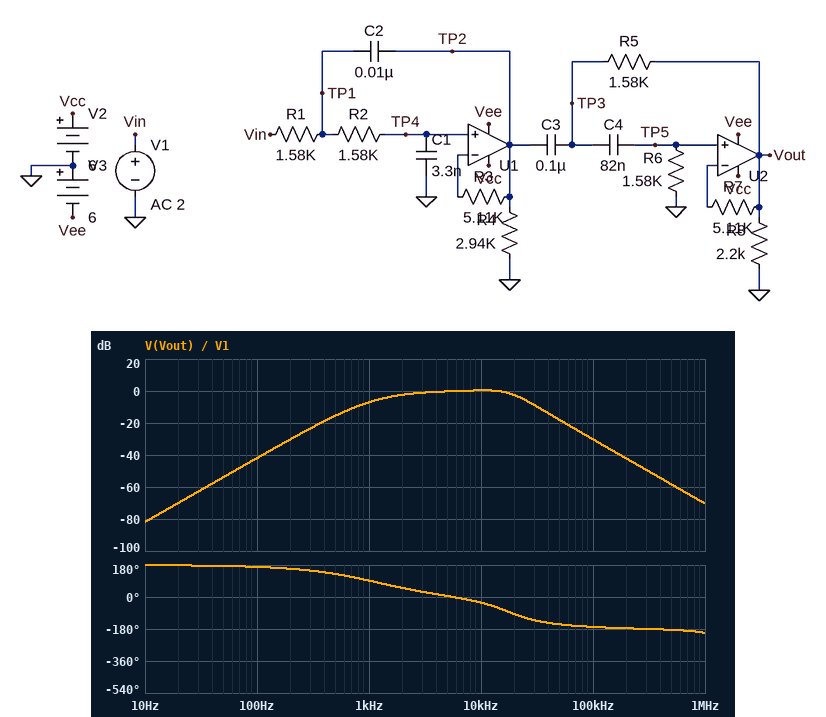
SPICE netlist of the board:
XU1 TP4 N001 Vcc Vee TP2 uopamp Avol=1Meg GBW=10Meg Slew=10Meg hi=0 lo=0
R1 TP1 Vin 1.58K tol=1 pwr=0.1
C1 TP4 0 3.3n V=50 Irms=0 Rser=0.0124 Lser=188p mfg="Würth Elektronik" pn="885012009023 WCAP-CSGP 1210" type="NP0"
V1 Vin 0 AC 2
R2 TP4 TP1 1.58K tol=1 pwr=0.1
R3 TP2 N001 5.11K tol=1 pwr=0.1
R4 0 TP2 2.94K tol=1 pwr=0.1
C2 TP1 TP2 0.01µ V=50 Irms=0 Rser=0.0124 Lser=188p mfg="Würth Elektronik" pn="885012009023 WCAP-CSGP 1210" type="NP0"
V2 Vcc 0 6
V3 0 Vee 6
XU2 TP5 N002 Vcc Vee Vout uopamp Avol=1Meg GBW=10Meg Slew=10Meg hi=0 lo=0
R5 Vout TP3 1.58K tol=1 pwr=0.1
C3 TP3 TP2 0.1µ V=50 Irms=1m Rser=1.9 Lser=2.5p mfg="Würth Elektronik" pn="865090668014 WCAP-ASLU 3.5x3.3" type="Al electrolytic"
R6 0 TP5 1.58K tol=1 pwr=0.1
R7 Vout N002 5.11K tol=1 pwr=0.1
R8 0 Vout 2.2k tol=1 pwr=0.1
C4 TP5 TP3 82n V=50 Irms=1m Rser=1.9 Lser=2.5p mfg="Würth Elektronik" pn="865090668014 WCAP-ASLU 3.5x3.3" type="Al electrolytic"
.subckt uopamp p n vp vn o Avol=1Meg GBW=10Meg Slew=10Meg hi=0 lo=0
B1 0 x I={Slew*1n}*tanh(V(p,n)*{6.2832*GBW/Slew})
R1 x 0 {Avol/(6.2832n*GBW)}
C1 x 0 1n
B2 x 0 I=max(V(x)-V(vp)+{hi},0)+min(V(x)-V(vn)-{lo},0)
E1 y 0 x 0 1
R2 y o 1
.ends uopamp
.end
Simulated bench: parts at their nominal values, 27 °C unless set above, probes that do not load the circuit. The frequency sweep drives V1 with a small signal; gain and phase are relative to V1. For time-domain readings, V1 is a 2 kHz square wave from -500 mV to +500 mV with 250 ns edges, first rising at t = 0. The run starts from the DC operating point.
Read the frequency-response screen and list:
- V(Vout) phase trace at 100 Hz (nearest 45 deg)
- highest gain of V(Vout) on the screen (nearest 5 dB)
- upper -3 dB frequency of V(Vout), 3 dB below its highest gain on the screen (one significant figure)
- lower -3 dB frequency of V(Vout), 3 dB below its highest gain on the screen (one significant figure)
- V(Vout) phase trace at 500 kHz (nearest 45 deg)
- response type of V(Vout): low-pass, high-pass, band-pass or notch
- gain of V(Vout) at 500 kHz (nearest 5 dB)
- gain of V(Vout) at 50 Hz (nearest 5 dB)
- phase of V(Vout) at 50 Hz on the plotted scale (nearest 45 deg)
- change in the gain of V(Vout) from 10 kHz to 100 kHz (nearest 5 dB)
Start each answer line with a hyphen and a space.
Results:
- 180 deg
- 0 dB
- 20 kHz
- 2 kHz
- -180 deg
- band-pass
- -60 dB
- -55 dB
- 180 deg
- -30 dB
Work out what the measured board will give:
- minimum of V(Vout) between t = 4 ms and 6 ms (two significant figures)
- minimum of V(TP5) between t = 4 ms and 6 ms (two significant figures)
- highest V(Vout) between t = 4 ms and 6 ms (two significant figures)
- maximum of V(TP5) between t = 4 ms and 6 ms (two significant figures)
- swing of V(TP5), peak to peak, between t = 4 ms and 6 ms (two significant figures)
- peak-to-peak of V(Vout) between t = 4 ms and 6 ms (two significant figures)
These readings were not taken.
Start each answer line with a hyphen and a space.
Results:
- -950 mV
- -950 mV
- 950 mV
- 950 mV
- 1.9 V
- 1.9 V
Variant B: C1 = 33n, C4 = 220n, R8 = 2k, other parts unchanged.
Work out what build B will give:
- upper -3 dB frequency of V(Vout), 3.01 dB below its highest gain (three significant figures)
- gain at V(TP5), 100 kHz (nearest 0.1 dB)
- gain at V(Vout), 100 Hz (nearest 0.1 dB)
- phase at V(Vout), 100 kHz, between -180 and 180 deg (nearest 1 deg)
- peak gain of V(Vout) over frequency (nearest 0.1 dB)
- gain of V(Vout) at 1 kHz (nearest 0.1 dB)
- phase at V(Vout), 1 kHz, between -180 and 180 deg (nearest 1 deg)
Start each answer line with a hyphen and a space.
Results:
- 3.34 kHz
- -50.4 dB
- -33.5 dB
- -169 deg
- -4.6 dB
- -5.2 dB
- 36 deg
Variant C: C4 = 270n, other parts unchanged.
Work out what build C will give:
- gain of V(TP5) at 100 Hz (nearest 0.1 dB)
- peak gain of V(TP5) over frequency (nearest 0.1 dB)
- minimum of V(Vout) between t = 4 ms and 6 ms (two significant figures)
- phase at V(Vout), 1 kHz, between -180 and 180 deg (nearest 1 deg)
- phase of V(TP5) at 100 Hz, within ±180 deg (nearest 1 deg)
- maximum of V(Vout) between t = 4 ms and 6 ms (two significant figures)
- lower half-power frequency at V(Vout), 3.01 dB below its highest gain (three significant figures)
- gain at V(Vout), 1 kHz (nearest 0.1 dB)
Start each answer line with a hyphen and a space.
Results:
- -31.8 dB
- 0.5 dB
- -910 mV
- 62 deg
- 159 deg
- 910 mV
- 1.25 kHz
- -3.6 dB
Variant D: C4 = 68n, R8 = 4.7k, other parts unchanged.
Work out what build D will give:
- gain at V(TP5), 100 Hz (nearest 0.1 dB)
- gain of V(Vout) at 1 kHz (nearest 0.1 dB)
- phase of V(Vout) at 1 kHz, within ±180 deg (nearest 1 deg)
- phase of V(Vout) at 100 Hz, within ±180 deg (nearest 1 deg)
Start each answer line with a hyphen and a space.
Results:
- -43.5 dB
- -8.1 dB
- 97 deg
- 170 deg
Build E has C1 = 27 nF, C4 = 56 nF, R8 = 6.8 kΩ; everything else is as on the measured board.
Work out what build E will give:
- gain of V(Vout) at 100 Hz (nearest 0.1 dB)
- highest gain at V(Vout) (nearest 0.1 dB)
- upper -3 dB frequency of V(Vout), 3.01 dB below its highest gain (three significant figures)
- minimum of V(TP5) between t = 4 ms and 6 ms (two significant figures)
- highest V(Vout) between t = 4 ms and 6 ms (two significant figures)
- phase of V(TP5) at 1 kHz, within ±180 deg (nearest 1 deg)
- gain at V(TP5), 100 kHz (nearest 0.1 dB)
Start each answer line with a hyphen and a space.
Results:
- -45.2 dB
- -6.4 dB
- 5.03 kHz
- -340 mV
- 340 mV
- 77 deg
- -48.7 dB
